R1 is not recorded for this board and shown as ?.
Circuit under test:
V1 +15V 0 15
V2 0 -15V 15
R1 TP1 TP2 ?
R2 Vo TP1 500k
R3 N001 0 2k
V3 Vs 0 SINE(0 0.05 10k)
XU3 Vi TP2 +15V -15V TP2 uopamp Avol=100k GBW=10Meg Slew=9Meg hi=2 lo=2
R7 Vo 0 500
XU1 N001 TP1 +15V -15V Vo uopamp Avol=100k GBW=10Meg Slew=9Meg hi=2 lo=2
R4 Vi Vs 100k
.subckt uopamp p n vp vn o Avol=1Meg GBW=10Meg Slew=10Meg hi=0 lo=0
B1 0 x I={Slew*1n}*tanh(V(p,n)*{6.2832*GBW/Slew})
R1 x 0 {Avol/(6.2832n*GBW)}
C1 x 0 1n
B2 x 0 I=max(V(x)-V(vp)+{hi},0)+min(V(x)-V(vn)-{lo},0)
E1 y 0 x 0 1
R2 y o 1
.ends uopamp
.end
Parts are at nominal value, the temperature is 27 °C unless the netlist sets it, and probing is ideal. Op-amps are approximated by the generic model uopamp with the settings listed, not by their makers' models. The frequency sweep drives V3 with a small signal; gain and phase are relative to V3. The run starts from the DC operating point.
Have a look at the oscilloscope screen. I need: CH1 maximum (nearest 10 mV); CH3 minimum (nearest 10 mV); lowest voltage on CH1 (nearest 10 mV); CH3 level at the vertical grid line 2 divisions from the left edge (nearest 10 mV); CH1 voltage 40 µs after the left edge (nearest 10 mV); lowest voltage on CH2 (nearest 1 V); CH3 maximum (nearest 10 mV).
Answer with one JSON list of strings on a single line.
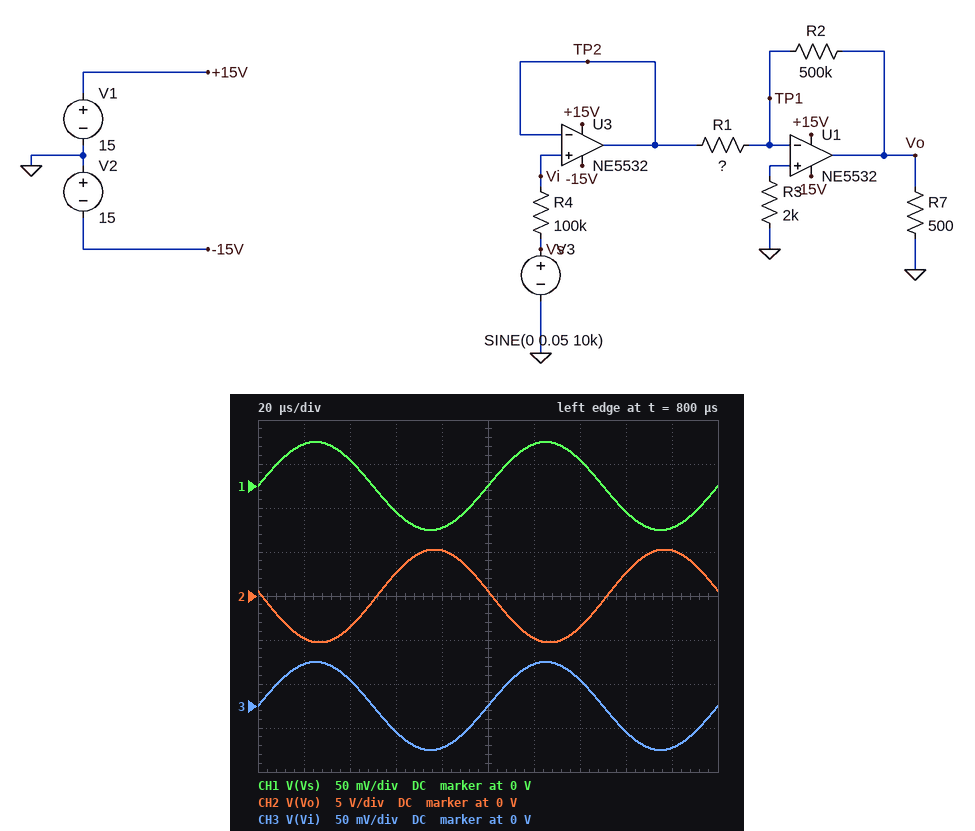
["50 mV", "-50 mV", "-50 mV", "30 mV", "30 mV", "-5 V", "50 mV"]
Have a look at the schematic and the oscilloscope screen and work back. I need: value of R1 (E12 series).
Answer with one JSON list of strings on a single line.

["4.7 kΩ"]
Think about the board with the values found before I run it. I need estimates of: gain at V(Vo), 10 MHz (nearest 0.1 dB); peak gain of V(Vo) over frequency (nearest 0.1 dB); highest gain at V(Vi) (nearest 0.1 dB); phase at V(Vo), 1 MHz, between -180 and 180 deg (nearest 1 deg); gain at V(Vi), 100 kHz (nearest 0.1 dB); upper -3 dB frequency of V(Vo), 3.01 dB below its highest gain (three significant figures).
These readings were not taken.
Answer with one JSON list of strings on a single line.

["-3.1 dB", "40.5 dB", "0 dB", "90 deg", "0 dB", "93.0 kHz"]
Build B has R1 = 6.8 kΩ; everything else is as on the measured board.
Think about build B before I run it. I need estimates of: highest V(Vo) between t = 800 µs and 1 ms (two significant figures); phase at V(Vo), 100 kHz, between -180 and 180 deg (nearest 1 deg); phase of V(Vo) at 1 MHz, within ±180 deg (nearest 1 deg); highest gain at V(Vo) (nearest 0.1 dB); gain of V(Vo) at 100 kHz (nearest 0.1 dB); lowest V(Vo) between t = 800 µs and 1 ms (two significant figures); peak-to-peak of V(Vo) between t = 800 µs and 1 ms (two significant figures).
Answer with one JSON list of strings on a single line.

["3.7 V", "143 deg", "92 deg", "37.3 dB", "35.4 dB", "-3.7 V", "7.3 V"]
